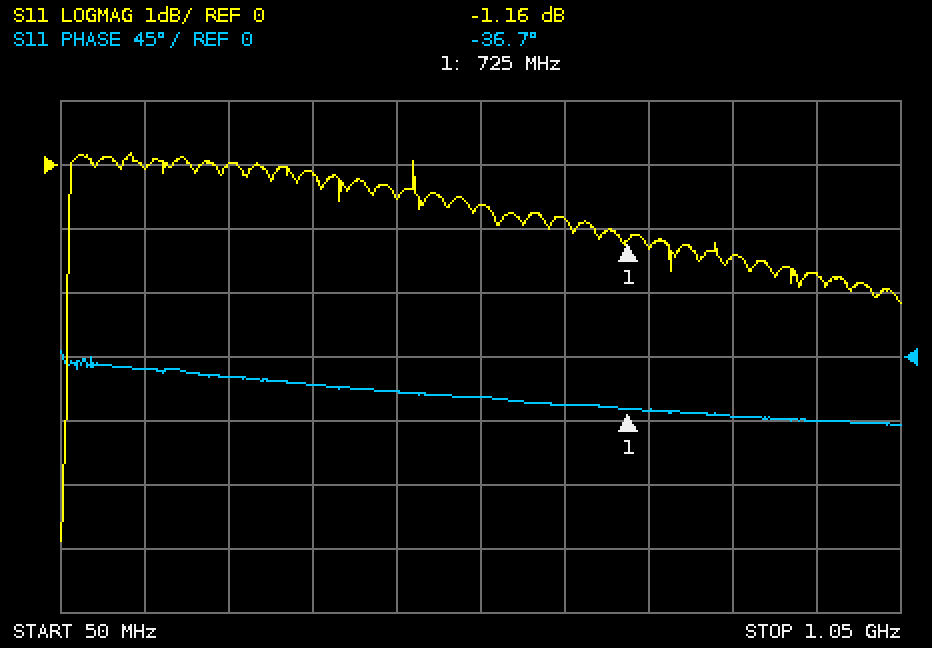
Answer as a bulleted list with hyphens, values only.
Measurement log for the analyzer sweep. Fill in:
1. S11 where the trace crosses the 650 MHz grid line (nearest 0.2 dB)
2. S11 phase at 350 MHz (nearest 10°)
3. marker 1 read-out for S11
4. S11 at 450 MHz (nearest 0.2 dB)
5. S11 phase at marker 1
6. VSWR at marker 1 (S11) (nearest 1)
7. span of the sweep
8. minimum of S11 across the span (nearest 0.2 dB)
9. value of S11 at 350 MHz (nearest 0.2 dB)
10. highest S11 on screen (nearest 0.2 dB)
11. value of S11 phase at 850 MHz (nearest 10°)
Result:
- -0.8 dB
- -20°
- -1.16 dB
- -0.6 dB
- -36.7°
- 15
- 1 GHz
- -5.8 dB
- -0.2 dB
- 0.2 dB
- -40°
